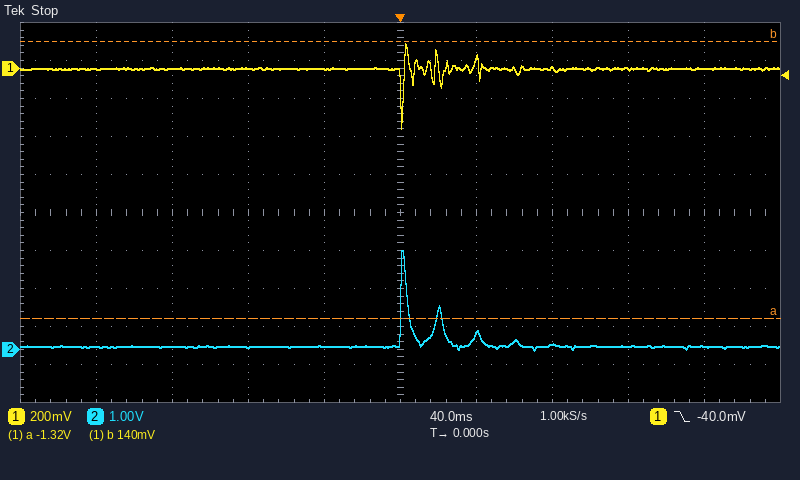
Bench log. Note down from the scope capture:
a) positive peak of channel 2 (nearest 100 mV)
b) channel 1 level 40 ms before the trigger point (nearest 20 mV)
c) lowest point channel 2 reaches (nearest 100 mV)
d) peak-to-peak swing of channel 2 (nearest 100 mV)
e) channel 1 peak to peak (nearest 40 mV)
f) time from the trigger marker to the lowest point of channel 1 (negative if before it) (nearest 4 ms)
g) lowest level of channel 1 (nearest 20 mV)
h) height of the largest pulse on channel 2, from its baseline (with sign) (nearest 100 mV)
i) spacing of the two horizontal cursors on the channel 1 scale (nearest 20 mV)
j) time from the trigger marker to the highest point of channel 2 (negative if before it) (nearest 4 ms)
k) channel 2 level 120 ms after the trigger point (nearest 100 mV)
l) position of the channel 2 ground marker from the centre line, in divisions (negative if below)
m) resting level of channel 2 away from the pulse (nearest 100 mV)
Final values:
2.6 V
0 mV
0.0 V
2.6 V
440 mV
0 ms
-320 mV
+2.5 V
1.46 V
0 ms
100 mV
-3.6 div
100 mV
